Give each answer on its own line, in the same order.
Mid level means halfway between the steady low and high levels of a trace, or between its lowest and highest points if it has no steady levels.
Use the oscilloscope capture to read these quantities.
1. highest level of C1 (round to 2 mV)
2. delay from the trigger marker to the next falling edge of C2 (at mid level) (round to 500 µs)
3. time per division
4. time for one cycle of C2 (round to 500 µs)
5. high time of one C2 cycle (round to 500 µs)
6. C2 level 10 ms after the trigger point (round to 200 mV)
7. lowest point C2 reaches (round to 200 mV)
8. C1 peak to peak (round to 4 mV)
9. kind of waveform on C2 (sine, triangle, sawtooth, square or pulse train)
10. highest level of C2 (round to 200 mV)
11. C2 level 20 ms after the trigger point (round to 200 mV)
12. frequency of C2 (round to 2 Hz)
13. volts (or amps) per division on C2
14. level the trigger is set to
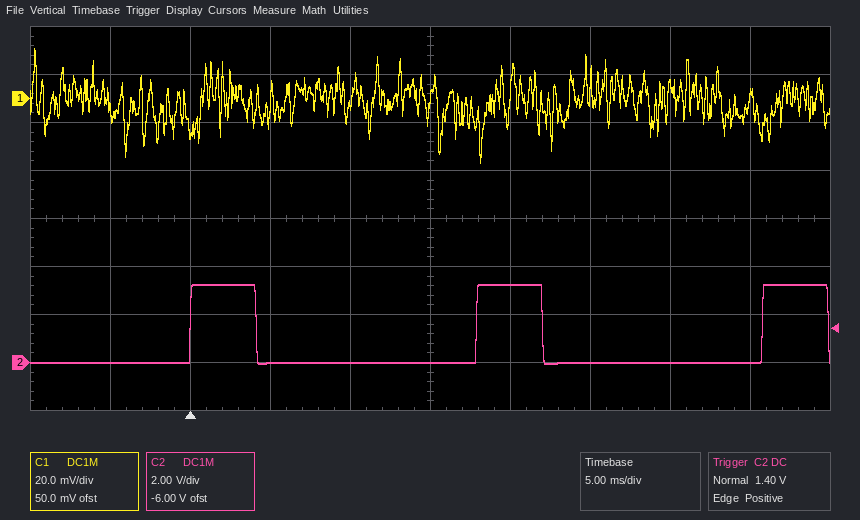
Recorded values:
20 mV
4.0 ms
5 ms
18.0 ms
4.0 ms
0.0 V
0.0 V
48 mV
pulse train
3.2 V
3.2 V
56 Hz
2 V
1.40 V
